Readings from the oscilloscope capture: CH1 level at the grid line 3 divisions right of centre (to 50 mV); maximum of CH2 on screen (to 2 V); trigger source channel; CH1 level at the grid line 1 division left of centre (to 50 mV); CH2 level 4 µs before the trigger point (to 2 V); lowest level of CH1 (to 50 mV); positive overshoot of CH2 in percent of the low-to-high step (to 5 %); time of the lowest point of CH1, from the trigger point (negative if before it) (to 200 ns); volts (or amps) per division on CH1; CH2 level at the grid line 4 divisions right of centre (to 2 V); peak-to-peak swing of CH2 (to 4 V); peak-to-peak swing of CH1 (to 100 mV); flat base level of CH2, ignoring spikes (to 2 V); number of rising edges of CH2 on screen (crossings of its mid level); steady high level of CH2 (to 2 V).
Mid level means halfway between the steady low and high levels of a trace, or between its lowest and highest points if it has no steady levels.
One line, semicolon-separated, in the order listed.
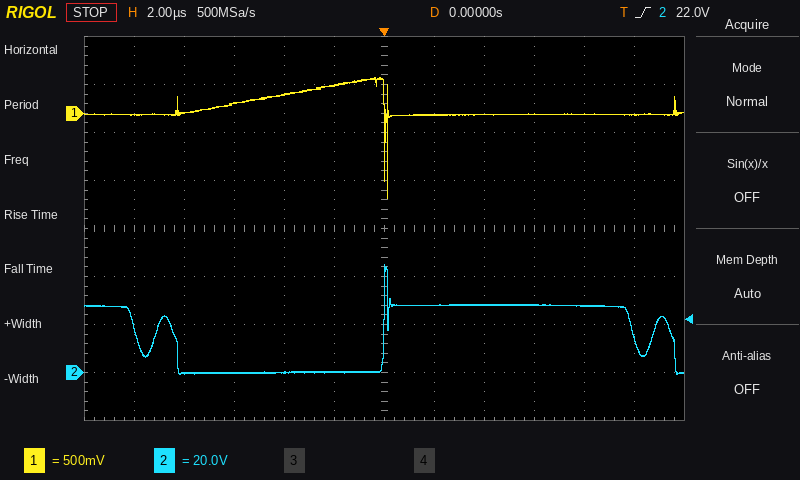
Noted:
0 mV; 44 V; CH2; 300 mV; 0 V; -900 mV; 60 %; +200 ns; 500 mV; 28 V; 44 V; 1.30 V; 0 V; 3; 28 V
